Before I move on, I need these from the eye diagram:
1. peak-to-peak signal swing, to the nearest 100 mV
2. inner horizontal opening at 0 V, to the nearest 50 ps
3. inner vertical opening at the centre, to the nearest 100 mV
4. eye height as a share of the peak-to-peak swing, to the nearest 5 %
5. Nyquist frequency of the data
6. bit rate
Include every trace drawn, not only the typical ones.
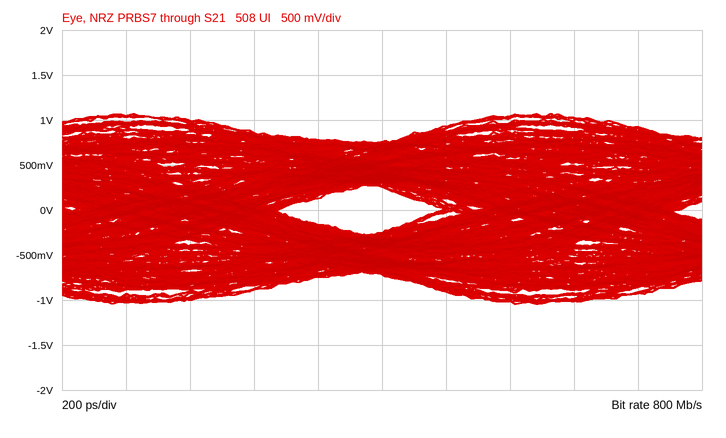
2.1 V
500 ps
500 mV
25 %
400 MHz
800 Mb/s
